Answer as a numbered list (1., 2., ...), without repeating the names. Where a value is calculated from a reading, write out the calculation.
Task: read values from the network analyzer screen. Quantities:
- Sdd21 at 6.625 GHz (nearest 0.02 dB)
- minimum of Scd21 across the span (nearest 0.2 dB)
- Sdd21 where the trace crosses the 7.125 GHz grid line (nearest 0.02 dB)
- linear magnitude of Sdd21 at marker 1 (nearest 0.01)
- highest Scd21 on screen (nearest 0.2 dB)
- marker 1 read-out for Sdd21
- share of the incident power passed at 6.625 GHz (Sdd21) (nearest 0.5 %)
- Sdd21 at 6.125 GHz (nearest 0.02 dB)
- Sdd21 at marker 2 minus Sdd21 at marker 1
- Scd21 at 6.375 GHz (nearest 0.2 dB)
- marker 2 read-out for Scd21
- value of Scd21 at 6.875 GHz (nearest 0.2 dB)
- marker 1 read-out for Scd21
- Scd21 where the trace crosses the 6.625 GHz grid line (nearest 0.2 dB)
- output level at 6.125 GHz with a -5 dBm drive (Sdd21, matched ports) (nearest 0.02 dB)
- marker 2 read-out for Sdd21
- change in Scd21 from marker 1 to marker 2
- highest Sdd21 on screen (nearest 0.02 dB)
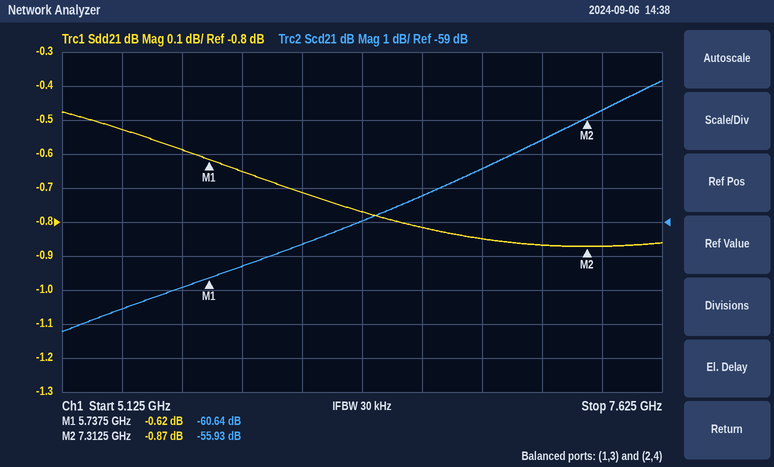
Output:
1. -0.82 dB
2. -62.2 dB
3. -0.86 dB
4. 10^(-0.62/20) ≈ 0.93
5. -54.8 dB
6. -0.62 dB
7. 10^(-0.82/10) ≈ 82.8 %, so 83.0 % to the nearest 0.5 %
8. -0.72 dB
9. -0.87 − (-0.62) = -0.25 dB
10. -59.0 dB
11. -55.93 dB
12. -57.4 dB
13. -60.64 dB
14. -58.2 dB
15. -5 dBm + (-0.72 dB) = -5.72 dBm
16. -0.87 dB
17. -55.93 − (-60.64) = 4.71 dB
18. -0.48 dB
